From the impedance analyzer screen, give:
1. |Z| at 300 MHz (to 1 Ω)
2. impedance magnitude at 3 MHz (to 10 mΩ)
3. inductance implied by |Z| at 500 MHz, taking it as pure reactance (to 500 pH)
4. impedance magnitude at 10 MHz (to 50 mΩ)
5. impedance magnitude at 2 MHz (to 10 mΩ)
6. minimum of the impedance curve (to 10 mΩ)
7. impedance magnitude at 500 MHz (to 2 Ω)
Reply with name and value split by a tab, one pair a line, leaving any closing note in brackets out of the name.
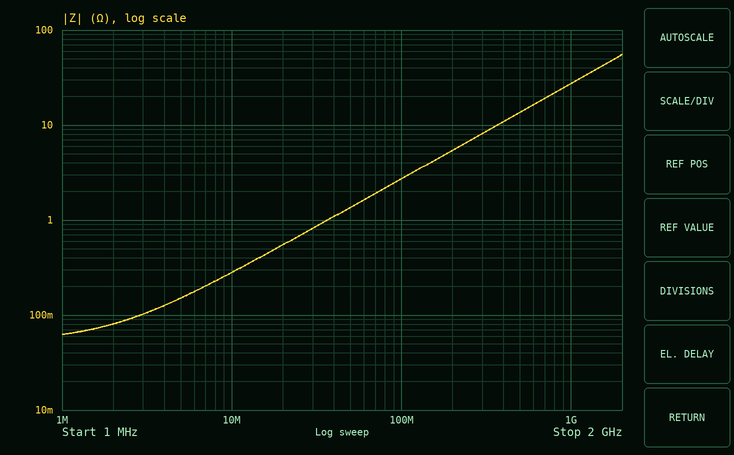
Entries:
|Z| at 300 MHz	8 Ω
impedance magnitude at 3 MHz	100 mΩ
inductance implied by |Z| at 500 MHz, taking it as pure reactance	4.5 nH
impedance magnitude at 10 MHz	300 mΩ
impedance magnitude at 2 MHz	80 mΩ
minimum of the impedance curve	60 mΩ
impedance magnitude at 500 MHz	14 Ω
